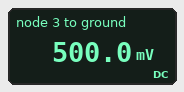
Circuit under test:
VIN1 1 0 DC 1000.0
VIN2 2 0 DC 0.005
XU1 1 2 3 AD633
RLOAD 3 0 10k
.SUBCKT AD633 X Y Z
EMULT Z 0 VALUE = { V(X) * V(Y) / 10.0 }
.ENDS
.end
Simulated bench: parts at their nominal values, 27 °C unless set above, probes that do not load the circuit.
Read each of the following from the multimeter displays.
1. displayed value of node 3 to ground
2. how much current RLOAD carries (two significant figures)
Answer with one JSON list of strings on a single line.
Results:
["500.0 mV", "50 µA"]
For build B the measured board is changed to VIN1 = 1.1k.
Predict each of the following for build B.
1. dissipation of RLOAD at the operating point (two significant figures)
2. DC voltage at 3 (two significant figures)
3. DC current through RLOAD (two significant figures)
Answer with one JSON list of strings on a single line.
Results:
["30 µW", "550 mV", "55 µA"]
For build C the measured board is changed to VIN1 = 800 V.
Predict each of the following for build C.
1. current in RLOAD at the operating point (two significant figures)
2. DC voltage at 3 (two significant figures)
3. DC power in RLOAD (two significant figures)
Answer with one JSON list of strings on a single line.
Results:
["40 µA", "400 mV", "16 µW"]
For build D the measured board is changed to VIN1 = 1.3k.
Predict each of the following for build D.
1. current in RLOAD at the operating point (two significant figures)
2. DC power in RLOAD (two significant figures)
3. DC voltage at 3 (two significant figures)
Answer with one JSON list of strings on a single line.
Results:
["65 µA", "42 µW", "650 mV"]
